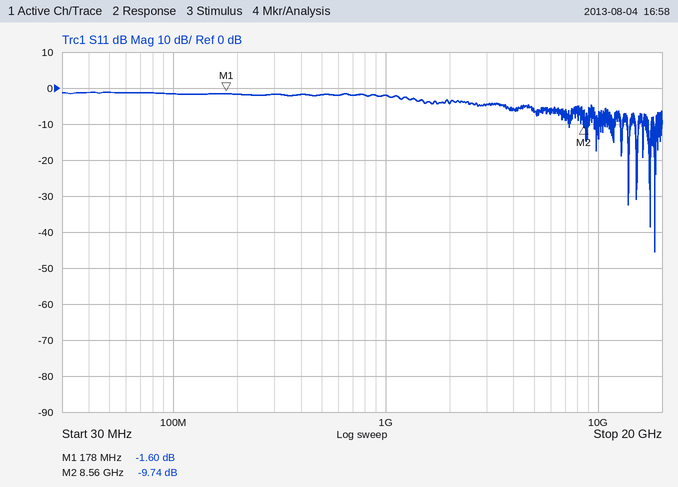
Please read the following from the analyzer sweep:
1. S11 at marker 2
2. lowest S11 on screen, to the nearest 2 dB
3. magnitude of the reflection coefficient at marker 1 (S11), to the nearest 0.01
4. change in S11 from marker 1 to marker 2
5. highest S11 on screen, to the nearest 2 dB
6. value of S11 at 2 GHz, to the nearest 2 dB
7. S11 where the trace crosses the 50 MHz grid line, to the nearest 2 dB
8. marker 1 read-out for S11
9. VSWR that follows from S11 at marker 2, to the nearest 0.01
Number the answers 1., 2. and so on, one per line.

1. -9.74 dB
2. -46 dB
3. 0.83
4. -8.14 dB
5. -2 dB
6. -4 dB
7. -2 dB
8. -1.60 dB
9. 1.97
